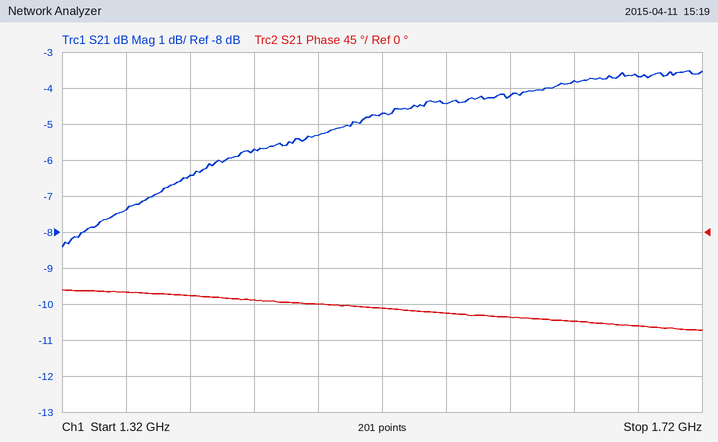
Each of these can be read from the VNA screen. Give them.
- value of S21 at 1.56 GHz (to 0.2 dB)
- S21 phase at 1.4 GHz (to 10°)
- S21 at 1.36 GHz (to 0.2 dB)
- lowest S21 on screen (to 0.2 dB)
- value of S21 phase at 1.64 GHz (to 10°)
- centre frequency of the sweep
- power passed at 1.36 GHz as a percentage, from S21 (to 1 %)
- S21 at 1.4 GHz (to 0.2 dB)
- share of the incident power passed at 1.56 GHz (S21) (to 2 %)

-4.4 dB
-80°
-7.4 dB
-8.4 dB
-110°
1.52 GHz
18 %
-6.4 dB
36 %
